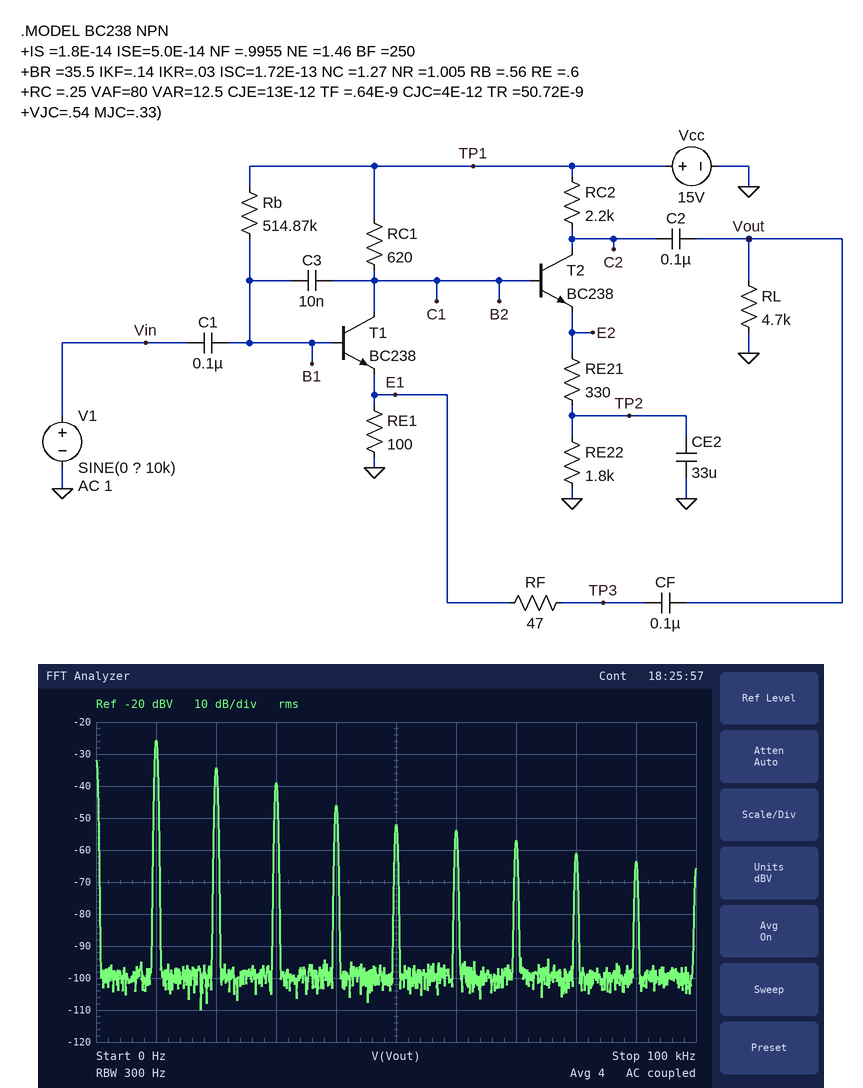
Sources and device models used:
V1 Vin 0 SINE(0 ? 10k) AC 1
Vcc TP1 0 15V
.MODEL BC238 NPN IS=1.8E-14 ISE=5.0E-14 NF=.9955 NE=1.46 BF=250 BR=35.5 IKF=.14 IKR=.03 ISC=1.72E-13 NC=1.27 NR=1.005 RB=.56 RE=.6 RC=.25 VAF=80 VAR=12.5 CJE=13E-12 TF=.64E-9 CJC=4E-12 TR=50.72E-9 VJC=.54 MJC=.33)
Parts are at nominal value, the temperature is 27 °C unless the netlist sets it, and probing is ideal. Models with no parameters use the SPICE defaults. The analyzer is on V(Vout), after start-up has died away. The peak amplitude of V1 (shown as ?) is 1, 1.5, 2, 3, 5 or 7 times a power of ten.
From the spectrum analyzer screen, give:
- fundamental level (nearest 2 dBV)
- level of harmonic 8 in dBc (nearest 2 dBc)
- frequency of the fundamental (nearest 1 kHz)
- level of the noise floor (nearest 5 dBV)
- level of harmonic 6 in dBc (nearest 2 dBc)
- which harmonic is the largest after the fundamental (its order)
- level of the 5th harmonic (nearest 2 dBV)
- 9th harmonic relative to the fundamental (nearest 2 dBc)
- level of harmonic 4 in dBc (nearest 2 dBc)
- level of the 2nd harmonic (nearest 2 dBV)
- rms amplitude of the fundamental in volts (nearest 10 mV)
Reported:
-26 dBV
-36 dBc
10 kHz
-100 dBV
-28 dBc
2
-52 dBV
-38 dBc
-20 dBc
-34 dBV
50 mV
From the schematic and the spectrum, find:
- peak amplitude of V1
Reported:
300 mV
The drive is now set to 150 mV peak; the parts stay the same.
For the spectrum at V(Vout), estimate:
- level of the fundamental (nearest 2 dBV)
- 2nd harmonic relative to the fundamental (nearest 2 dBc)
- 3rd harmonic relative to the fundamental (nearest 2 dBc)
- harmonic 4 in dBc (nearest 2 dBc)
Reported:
-28 dBV
-34 dBc
-42 dBc
-54 dBc
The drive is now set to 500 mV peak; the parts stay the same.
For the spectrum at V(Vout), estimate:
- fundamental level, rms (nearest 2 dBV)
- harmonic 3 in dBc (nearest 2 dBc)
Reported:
-26 dBV
-8 dBc
